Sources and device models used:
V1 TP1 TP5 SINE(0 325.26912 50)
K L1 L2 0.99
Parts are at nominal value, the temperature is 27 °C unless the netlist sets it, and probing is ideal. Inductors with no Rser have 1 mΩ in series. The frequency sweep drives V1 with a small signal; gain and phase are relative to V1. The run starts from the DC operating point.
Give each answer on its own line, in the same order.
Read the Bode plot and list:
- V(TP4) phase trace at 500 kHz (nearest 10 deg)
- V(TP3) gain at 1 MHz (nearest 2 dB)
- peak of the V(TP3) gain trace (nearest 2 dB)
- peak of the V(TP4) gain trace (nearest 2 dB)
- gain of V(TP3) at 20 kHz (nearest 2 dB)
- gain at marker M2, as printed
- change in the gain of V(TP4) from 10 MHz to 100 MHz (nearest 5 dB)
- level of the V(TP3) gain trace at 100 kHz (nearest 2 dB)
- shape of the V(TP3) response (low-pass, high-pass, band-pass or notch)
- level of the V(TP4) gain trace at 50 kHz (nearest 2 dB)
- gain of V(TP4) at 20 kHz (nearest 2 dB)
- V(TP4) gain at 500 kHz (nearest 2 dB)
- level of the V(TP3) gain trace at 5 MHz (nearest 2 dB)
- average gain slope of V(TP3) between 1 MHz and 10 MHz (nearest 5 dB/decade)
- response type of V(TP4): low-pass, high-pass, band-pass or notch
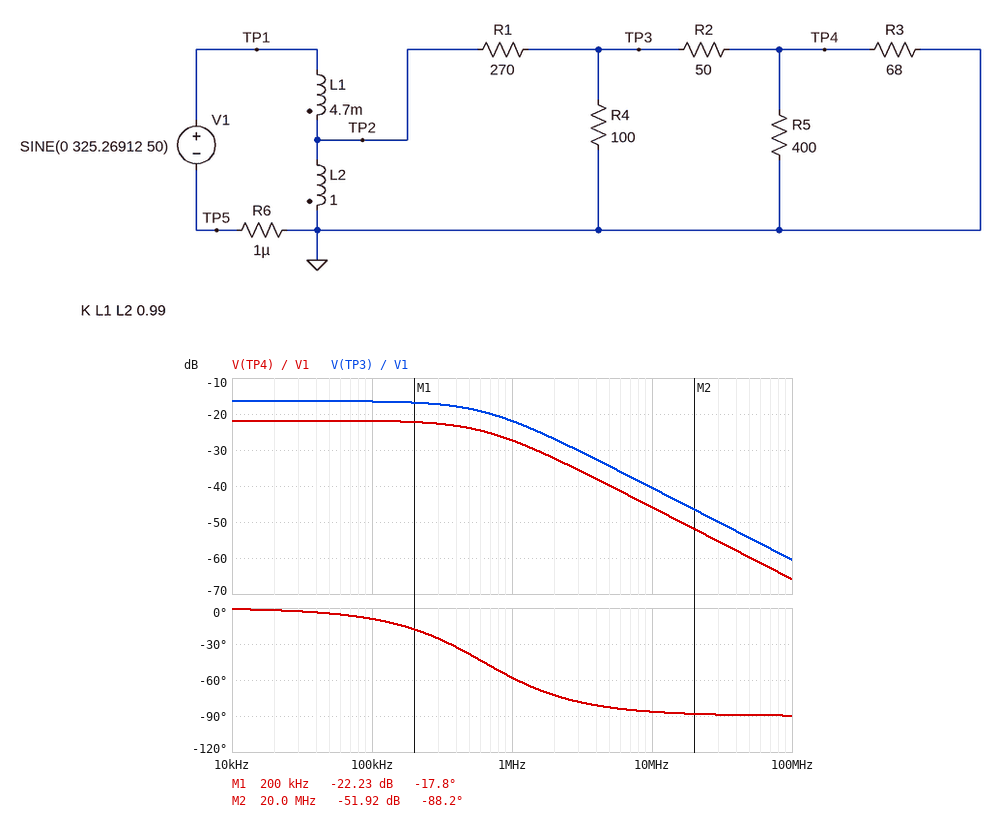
-40 deg
-22 dB
-16 dB
-22 dB
-16 dB
-51.92 dB
-20 dB
-16 dB
low-pass
-22 dB
-22 dB
-24 dB
-34 dB
-20 dB/decade
low-pass
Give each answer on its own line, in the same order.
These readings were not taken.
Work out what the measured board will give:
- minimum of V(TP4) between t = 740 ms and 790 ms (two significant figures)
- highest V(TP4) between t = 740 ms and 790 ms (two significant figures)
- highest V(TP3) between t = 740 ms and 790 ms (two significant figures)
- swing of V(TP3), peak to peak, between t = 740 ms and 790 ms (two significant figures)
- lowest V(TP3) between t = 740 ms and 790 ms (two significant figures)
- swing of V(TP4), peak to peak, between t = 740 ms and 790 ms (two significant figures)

-26 V
26 V
49 V
98 V
-49 V
53 V
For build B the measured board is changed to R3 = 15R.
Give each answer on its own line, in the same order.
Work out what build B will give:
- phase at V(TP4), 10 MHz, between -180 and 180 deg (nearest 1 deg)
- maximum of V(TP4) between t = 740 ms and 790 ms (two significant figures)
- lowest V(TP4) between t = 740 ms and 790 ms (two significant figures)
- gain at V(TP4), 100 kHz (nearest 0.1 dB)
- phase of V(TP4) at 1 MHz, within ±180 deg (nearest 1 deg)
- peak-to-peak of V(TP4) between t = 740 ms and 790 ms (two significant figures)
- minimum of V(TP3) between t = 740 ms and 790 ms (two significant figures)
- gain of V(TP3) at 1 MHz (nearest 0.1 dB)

-87 deg
8.7 V
-8.7 V
-31.6 dB
-59 deg
17 V
-39 V
-24.3 dB
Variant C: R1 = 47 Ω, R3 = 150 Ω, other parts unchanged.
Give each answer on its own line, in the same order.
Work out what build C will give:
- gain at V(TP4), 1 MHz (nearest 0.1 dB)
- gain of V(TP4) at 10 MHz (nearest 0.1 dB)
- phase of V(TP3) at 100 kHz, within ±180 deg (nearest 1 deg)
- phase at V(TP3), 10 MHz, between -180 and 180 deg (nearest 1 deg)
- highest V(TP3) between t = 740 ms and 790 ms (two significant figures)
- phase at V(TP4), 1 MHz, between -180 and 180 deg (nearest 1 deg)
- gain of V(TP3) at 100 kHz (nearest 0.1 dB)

-22.5 dB
-42.3 dB
-25 deg
-89 deg
170 V
-78 deg
-6.4 dB
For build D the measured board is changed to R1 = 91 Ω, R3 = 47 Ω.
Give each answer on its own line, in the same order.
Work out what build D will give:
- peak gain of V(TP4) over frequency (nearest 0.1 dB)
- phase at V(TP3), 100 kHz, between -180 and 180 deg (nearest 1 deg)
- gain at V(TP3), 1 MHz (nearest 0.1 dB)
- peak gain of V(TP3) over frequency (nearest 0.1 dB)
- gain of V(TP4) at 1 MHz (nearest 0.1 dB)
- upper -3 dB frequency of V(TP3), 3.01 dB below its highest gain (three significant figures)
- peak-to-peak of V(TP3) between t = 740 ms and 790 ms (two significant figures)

-16.6 dB
-20 deg
-21.5 dB
-9.8 dB
-28.3 dB
270 kHz
210 V
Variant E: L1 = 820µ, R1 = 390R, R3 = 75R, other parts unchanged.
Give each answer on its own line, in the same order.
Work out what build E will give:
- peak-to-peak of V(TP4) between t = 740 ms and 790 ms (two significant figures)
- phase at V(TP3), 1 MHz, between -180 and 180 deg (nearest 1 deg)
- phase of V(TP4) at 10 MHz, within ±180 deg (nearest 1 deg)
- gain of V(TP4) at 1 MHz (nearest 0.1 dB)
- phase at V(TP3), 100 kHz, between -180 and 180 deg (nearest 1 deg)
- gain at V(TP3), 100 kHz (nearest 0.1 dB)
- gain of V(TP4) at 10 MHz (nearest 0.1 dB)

42 V
-12 deg
-65 deg
-23.9 dB
-1 deg
-18.7 dB
-31.4 dB
